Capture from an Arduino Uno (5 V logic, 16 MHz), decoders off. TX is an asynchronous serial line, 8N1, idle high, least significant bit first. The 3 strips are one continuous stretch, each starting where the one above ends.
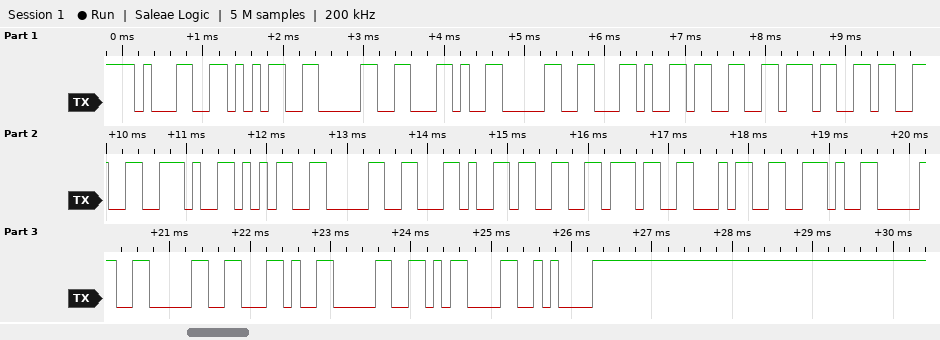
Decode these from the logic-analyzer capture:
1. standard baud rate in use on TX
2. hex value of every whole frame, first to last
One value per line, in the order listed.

9600 baud
31 35 30 2C 30 2C 33 37 33 2E 35 30 2C 33 37 34 2E 30 30 2C 30 0D 0A
